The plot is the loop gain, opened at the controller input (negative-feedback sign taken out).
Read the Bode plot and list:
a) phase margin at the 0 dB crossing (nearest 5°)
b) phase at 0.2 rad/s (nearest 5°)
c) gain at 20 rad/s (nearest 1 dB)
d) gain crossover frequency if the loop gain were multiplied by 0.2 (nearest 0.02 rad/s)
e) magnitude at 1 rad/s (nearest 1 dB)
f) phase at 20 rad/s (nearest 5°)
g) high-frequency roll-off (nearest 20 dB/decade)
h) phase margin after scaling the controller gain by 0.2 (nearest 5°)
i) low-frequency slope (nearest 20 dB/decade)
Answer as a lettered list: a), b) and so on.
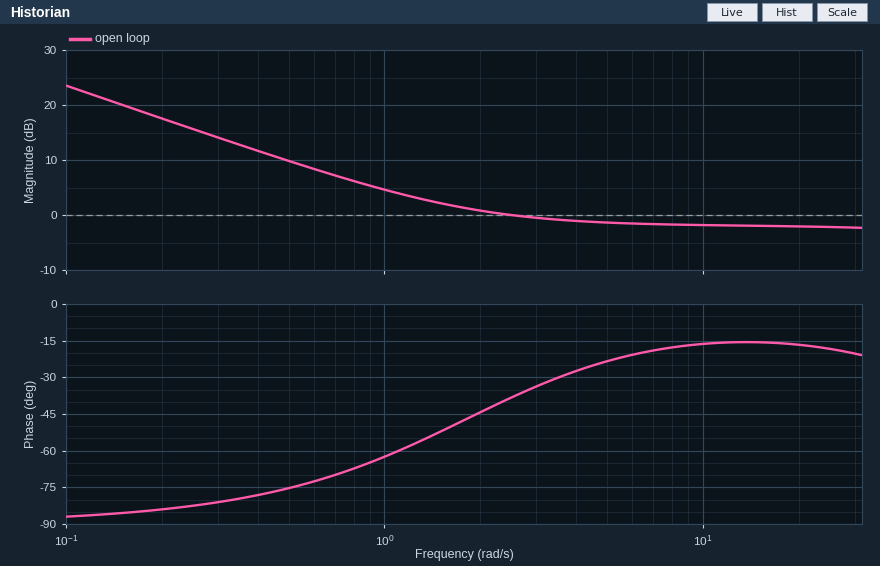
a) 140°
b) -85°
c) -2 dB
d) 0.30 rad/s
e) 5 dB
f) -15°
g) 0 dB/decade
h) 100°
i) -20 dB/decade
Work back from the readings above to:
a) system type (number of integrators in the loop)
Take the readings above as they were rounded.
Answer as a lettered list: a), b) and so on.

a) 1
